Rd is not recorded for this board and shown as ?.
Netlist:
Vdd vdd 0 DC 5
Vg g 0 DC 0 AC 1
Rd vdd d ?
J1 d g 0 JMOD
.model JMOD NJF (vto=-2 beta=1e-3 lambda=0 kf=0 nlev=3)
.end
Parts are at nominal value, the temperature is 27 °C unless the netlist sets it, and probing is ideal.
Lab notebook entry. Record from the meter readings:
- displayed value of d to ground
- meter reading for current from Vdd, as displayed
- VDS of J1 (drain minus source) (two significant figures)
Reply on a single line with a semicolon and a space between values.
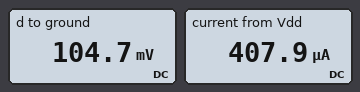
104.7 mV; 407.9 µA; 100 mV
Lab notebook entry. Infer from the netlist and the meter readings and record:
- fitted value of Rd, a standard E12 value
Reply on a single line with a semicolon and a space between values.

12 kΩ
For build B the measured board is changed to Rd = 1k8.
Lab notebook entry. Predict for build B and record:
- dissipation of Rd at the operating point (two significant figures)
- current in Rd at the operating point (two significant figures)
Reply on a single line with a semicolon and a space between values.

10 mW; 2.4 mA
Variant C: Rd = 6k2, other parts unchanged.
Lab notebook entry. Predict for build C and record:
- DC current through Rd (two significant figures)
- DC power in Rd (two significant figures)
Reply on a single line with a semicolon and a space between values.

770 µA; 3.7 mW
